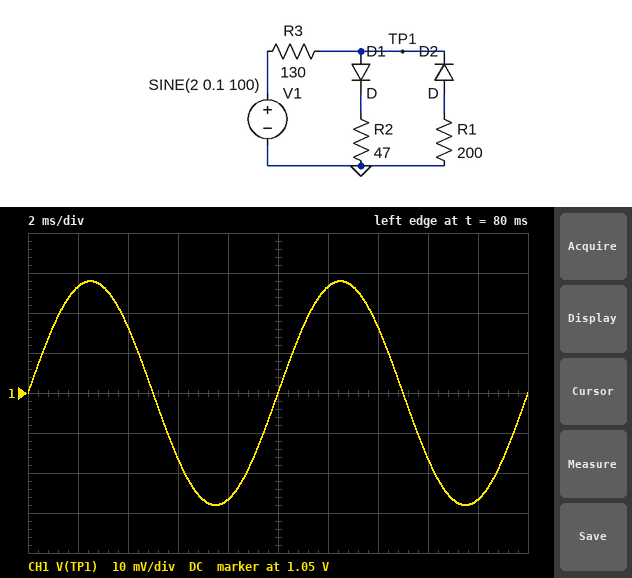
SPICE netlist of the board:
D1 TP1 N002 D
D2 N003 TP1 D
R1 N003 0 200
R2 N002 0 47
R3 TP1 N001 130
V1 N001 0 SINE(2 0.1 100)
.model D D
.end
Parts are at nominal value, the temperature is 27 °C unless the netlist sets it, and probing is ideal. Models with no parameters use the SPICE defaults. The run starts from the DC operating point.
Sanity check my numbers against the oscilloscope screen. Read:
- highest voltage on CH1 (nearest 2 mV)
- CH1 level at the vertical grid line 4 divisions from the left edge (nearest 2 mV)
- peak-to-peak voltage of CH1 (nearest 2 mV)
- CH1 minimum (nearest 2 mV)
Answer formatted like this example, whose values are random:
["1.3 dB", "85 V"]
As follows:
["1.078 V", "1.024 V", "56 mV", "1.022 V"]
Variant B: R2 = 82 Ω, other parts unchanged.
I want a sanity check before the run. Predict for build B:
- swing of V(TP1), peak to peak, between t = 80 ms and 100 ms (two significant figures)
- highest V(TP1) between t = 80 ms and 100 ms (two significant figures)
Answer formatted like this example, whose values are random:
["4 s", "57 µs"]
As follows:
["80 mV", "1.2 V"]
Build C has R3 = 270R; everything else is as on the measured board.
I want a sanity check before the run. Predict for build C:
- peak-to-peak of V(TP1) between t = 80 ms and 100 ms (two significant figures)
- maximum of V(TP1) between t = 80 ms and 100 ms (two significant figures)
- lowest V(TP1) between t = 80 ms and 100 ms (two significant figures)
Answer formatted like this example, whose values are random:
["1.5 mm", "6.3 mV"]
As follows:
["33 mV", "900 mV", "870 mV"]
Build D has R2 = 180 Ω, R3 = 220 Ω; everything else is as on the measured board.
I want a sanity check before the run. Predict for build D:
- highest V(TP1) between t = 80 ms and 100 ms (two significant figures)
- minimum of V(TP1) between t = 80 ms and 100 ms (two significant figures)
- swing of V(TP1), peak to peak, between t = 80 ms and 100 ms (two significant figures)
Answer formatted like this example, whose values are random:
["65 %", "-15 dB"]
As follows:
["1.3 V", "1.2 V", "92 mV"]
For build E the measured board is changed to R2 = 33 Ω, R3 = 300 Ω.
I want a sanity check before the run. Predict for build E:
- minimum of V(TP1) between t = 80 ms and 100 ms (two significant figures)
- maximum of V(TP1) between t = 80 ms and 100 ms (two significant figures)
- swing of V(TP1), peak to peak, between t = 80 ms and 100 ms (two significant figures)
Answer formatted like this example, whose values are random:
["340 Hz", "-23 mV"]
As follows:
["810 mV", "830 mV", "23 mV"]
